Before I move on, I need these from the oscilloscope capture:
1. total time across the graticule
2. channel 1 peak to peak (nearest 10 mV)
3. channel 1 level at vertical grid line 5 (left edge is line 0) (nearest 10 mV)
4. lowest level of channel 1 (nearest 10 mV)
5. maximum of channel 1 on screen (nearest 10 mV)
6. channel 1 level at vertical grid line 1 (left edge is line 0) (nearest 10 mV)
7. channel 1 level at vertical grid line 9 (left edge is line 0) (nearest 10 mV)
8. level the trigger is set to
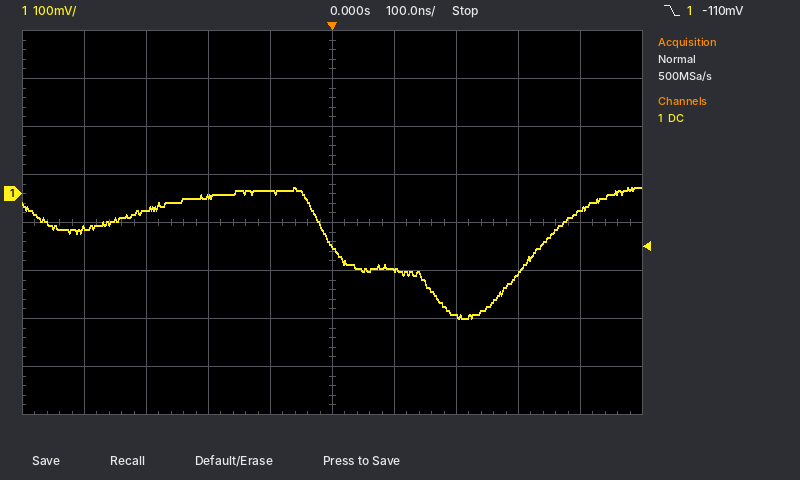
1 µs
270 mV
-110 mV
-260 mV
10 mV
-70 mV
-30 mV
-110 mV
